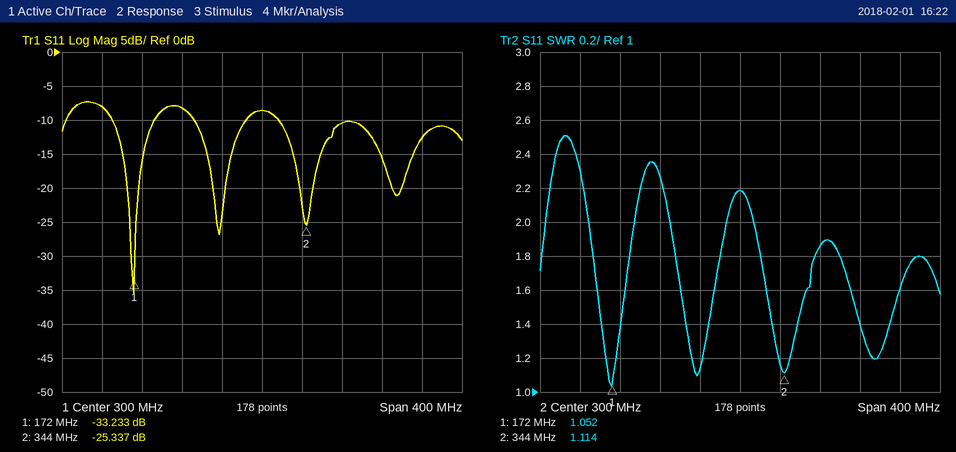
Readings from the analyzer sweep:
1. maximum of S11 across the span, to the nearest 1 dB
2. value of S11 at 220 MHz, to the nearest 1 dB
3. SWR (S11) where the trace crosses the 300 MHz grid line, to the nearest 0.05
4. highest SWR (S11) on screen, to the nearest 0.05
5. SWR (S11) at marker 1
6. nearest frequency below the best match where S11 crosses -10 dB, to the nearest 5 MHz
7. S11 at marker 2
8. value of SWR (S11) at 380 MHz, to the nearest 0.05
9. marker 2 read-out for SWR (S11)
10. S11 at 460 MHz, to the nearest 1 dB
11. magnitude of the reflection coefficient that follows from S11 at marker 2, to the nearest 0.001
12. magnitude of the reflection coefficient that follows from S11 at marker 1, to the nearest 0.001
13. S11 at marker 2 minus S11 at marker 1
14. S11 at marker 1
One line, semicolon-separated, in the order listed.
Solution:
-7 dB; -8 dB; 2.20; 2.50; 1.052; 150 MHz; -25.337 dB; 1.85; 1.114; -13 dB; 0.054; 0.022; 7.896 dB; -33.233 dB
